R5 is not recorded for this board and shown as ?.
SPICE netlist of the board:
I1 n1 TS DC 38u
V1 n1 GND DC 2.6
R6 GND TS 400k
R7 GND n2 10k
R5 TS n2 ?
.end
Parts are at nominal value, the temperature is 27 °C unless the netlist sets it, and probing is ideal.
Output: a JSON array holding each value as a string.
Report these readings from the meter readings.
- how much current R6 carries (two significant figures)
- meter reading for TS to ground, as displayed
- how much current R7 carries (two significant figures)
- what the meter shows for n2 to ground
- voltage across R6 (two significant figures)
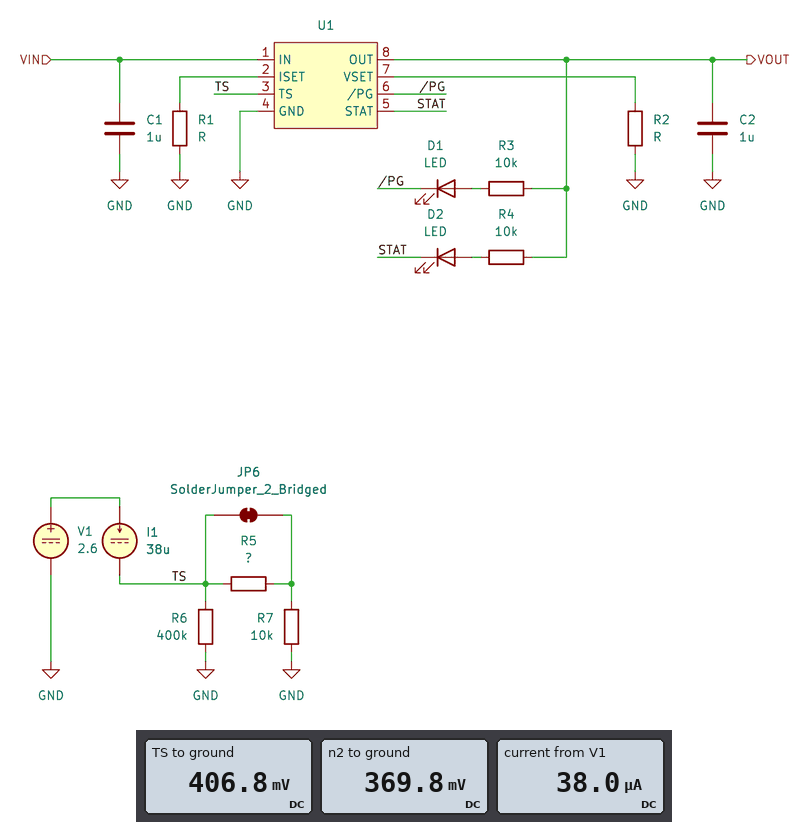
["1.0 µA", "406.8 mV", "37 µA", "369.8 mV", "410 mV"]
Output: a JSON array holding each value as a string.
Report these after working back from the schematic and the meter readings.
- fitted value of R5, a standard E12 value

["1 kΩ"]
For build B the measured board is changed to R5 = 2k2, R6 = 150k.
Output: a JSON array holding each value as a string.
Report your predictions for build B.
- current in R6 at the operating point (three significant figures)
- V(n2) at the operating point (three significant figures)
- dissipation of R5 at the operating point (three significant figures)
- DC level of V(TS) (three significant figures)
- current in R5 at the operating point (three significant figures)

["2.86 µA", "351 mV", "2.72 µW", "429 mV", "35.1 µA"]
